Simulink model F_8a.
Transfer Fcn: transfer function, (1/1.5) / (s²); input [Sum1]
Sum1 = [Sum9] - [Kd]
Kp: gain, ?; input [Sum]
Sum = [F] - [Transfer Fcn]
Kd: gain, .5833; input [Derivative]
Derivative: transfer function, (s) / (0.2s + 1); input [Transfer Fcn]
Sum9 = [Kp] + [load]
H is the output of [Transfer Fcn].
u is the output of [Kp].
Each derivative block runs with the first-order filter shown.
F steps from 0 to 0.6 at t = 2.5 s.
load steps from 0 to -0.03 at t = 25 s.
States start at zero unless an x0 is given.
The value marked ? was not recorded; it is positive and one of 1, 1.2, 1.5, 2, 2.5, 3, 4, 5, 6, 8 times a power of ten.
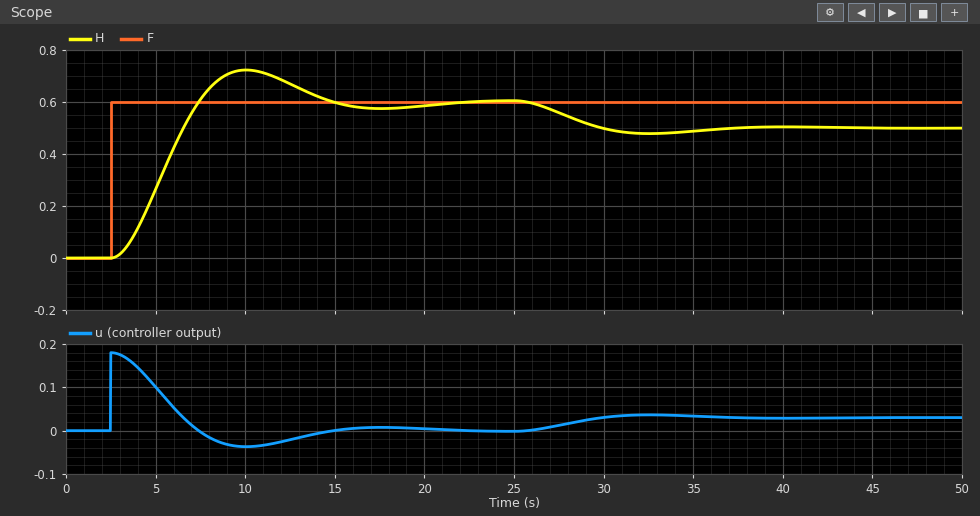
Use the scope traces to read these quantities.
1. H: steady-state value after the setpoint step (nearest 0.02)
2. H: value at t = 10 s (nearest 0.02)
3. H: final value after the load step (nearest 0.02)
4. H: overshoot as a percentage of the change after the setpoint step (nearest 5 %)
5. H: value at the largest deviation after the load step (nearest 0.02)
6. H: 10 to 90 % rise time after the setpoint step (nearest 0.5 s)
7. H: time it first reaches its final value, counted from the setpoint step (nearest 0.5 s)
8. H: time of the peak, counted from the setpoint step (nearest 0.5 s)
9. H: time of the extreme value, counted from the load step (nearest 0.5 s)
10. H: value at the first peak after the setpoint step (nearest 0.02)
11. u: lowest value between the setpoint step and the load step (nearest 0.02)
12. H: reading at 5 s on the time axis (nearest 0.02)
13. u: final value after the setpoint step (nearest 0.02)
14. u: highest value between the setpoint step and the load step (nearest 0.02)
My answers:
0.60
0.72
0.50
20 %
0.48
3.5 s
5.0 s
7.5 s
7.5 s
0.72
-0.04
0.26
0.00
0.18
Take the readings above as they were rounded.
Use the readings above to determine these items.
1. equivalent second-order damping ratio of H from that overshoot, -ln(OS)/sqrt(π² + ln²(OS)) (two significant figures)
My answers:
0.46
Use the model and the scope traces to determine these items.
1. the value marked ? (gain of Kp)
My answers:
0.3
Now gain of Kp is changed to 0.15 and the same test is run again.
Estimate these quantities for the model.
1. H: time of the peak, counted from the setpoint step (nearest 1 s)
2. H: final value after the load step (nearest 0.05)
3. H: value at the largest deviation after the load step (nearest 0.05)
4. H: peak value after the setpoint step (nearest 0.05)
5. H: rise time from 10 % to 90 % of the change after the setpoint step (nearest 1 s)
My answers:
12 s
0.40
0.40
0.65
6 s
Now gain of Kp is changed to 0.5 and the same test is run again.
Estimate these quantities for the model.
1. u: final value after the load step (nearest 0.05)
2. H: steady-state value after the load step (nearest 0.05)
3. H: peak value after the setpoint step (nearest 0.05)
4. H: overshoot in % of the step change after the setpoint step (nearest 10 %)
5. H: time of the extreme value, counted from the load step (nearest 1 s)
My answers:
0.05
0.55
0.80
30 %
6 s
